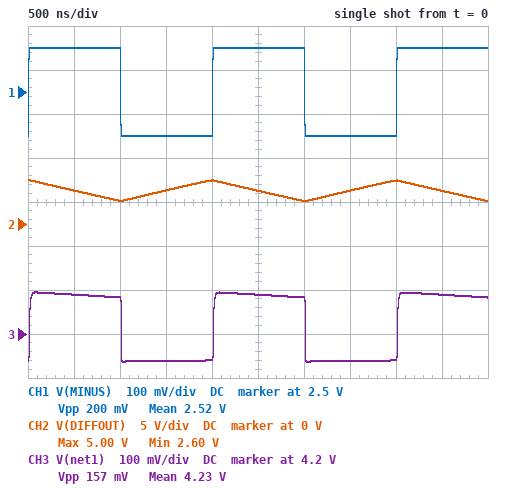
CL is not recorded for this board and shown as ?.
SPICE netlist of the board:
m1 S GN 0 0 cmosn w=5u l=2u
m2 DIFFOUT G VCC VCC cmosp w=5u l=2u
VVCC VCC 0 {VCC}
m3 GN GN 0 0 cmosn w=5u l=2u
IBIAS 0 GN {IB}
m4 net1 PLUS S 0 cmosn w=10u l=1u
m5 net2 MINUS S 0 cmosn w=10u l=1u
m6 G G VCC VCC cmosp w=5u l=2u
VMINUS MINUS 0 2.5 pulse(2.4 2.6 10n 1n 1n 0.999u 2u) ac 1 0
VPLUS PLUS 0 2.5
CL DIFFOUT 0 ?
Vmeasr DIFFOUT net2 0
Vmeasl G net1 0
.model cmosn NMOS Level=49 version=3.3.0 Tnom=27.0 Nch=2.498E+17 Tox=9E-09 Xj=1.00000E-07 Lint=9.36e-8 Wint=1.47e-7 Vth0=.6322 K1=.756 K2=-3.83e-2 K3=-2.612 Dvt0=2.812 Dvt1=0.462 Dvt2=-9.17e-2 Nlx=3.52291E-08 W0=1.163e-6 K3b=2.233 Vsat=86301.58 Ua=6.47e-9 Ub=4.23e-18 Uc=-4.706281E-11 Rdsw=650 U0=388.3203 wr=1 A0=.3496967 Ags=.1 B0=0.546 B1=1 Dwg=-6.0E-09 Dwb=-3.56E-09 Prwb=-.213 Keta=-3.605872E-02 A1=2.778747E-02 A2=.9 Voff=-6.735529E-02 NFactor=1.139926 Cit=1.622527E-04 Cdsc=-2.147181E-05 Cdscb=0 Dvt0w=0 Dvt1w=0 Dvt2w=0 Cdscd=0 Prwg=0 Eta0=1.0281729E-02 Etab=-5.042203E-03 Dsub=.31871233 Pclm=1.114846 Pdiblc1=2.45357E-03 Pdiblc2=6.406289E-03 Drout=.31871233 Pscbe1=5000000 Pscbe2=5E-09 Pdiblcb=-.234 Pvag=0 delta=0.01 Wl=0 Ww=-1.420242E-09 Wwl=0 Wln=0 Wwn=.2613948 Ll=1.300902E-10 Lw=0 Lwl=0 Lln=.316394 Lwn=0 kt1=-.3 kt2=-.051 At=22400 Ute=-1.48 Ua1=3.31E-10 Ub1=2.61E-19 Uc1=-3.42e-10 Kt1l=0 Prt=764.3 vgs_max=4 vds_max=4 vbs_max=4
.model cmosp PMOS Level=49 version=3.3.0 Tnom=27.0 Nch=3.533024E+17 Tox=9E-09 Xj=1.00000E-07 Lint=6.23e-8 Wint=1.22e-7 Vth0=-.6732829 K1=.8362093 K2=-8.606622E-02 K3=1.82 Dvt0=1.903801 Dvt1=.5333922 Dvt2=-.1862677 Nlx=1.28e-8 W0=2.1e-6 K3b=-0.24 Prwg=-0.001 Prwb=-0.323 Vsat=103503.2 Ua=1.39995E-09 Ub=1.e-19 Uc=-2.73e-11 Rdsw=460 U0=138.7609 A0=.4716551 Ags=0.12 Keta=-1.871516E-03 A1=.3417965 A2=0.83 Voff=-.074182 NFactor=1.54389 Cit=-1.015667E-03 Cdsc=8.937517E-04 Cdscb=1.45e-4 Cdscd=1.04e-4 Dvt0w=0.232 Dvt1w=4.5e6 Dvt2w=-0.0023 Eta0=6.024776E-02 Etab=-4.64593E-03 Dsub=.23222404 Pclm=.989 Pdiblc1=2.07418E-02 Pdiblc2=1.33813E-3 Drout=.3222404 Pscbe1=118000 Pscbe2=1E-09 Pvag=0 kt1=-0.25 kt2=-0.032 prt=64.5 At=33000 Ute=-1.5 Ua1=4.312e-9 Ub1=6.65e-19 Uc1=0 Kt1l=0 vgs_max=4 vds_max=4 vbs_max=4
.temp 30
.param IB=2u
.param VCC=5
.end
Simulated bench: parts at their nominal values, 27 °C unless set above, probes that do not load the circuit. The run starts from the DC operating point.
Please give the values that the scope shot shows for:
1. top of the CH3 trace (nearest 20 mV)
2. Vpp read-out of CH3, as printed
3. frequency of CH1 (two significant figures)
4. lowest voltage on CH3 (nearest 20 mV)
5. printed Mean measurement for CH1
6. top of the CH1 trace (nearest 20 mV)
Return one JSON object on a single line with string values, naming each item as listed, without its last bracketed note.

{"top of the CH3 trace": "4.30 V", "Vpp read-out of CH3, as printed": "157 mV", "frequency of CH1": "500 kHz", "lowest voltage on CH3": "4.14 V", "printed Mean measurement for CH1": "2.52 V", "top of the CH1 trace": "2.60 V"}
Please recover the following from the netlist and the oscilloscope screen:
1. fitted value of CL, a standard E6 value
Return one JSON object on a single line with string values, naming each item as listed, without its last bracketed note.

{"fitted value of CL, a standard E6 value": "680 fF"}
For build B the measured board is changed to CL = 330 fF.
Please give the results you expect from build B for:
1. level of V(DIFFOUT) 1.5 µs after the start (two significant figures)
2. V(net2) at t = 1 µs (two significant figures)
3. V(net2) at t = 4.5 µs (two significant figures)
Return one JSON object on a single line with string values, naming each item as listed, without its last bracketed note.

{"level of V(DIFFOUT) 1.5 µs after the start": "4.0 V", "V(net2) at t = 1 µs": "1.5 V", "V(net2) at t = 4.5 µs": "2.6 V"}
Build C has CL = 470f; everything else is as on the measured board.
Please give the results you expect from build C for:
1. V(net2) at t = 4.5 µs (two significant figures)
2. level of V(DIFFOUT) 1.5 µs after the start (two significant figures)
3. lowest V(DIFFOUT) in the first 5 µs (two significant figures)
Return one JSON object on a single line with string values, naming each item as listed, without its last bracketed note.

{"V(net2) at t = 4.5 µs": "3.3 V", "level of V(DIFFOUT) 1.5 µs after the start": "3.4 V", "lowest V(DIFFOUT) in the first 5 µs": "1.6 V"}
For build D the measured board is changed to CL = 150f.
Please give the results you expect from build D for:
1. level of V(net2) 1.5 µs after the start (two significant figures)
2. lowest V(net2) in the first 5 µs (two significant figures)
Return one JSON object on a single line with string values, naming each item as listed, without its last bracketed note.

{"level of V(net2) 1.5 µs after the start": "5.0 V", "lowest V(net2) in the first 5 µs": "1.5 V"}
